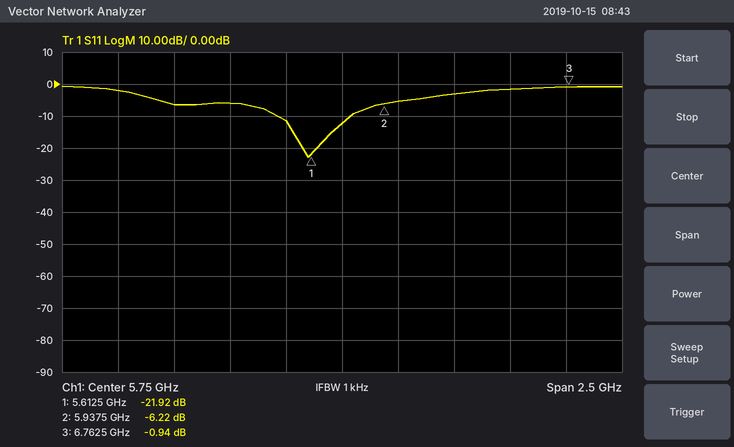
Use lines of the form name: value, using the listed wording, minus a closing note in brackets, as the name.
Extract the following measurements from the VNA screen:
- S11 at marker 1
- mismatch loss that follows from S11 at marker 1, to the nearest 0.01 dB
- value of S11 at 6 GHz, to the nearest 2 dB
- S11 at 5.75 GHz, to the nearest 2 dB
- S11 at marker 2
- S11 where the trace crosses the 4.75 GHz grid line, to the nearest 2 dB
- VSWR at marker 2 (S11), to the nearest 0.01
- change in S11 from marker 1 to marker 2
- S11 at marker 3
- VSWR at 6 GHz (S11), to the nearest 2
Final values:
S11 at marker 1: -21.92 dB
mismatch loss that follows from S11 at marker 1, to the nearest 0.01 dB: 0.03 dB
value of S11 at 6 GHz, to the nearest 2 dB: -6 dB
S11 at 5.75 GHz, to the nearest 2 dB: -12 dB
S11 at marker 2: -6.22 dB
S11 where the trace crosses the 4.75 GHz grid line, to the nearest 2 dB: -2 dB
VSWR at marker 2 (S11), to the nearest 0.01: 2.91
change in S11 from marker 1 to marker 2: 15.70 dB
S11 at marker 3: -0.94 dB
VSWR at 6 GHz (S11), to the nearest 2: 4
